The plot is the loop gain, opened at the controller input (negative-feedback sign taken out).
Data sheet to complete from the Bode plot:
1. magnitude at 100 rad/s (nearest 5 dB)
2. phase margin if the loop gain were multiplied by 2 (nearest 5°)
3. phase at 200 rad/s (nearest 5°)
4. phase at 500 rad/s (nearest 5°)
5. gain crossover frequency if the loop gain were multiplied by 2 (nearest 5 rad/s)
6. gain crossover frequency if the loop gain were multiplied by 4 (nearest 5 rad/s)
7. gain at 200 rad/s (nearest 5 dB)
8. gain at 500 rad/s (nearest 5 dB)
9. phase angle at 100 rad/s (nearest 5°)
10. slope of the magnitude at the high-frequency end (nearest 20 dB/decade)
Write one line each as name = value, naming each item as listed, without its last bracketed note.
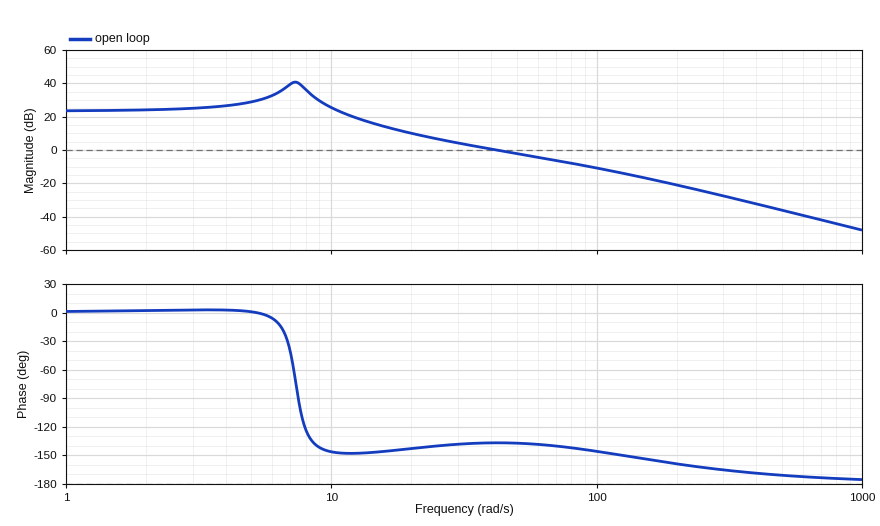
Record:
magnitude at 100 rad/s = -10 dB
phase margin if the loop gain were multiplied by 2 = 40°
phase at 200 rad/s = -160°
phase at 500 rad/s = -170°
gain crossover frequency if the loop gain were multiplied by 2 = 70 rad/s
gain crossover frequency if the loop gain were multiplied by 4 = 110 rad/s
gain at 200 rad/s = -20 dB
gain at 500 rad/s = -35 dB
phase angle at 100 rad/s = -145°
slope of the magnitude at the high-frequency end = -40 dB/decade
